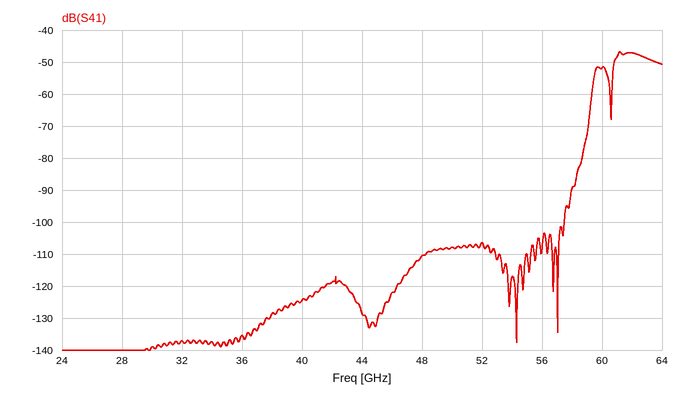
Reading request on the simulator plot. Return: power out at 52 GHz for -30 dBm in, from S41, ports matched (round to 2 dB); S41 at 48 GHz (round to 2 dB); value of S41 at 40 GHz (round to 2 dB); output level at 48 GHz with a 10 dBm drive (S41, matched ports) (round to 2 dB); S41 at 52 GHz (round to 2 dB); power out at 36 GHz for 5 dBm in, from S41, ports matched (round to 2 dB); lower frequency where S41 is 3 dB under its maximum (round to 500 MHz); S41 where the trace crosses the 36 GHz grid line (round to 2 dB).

-136 dBm
-110 dB
-124 dB
-100 dBm
-106 dB
-130 dBm
61.0 GHz
-136 dB
